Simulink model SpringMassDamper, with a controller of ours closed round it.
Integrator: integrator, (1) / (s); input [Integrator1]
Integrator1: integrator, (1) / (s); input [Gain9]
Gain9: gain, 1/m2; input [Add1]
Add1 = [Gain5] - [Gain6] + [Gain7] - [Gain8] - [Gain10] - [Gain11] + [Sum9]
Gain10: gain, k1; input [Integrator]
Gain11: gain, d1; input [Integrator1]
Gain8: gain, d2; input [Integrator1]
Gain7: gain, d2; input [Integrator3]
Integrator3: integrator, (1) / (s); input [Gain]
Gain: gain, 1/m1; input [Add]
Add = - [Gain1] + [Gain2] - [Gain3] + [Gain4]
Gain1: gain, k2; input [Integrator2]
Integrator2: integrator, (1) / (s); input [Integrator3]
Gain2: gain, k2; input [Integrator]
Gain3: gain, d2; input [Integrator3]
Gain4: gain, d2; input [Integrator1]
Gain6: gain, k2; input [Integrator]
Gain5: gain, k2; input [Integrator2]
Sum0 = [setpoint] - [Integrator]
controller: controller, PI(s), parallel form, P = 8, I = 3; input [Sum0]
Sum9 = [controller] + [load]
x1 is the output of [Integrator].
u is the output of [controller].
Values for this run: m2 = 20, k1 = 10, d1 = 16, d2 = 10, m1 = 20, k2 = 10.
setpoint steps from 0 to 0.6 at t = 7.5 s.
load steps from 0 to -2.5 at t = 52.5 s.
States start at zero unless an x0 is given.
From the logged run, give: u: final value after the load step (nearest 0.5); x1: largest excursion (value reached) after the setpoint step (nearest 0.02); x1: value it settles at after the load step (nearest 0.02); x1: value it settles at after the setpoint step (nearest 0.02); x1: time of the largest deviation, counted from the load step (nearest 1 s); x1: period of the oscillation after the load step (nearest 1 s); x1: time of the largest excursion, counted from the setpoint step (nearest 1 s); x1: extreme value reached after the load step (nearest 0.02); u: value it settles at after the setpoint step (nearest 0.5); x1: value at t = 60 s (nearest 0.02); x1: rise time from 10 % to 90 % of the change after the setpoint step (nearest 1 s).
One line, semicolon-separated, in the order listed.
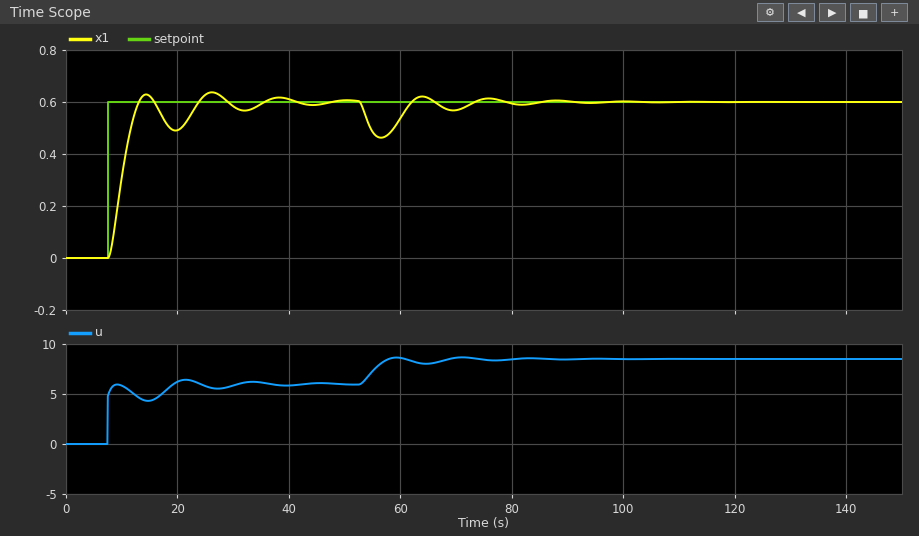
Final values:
8.5; 0.64; 0.60; 0.60; 4 s; 13 s; 19 s; 0.46; 6.0; 0.54; 4 s
